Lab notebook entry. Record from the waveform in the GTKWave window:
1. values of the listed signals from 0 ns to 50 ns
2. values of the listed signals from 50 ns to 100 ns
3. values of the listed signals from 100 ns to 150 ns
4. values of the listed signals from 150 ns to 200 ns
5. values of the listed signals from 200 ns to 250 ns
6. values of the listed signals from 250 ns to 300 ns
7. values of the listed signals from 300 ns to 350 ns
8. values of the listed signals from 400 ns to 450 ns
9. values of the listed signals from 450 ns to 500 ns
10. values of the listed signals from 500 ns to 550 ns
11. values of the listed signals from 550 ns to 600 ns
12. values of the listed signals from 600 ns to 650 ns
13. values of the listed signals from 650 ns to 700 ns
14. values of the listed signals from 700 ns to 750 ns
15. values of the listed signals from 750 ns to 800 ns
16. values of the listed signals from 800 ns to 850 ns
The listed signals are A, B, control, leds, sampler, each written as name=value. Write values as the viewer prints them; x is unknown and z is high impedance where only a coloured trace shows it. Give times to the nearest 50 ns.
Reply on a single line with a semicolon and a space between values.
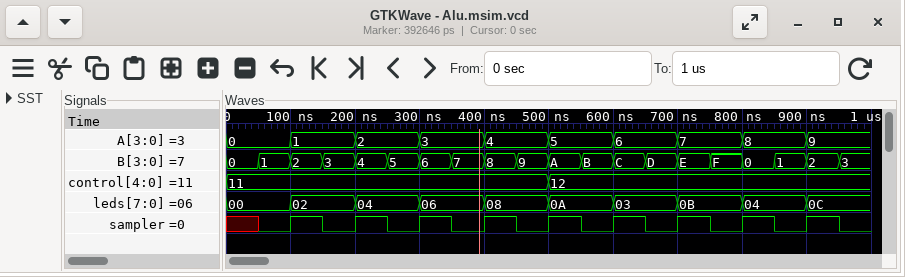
A=0, B=0, control=11, leds=00, sampler=x; A=0, B=1, control=11, leds=00, sampler=0; A=1, B=2, control=11, leds=02, sampler=1; A=1, B=3, control=11, leds=02, sampler=0; A=2, B=4, control=11, leds=04, sampler=1; A=2, B=5, control=11, leds=04, sampler=0; A=3, B=6, control=11, leds=06, sampler=1; A=4, B=8, control=11, leds=08, sampler=1; A=4, B=9, control=11, leds=08, sampler=0; A=5, B=A, control=12, leds=0A, sampler=1; A=5, B=B, control=12, leds=0A, sampler=0; A=6, B=C, control=12, leds=03, sampler=1; A=6, B=D, control=12, leds=03, sampler=0; A=7, B=E, control=12, leds=0B, sampler=1; A=7, B=F, control=12, leds=0B, sampler=0; A=8, B=0, control=12, leds=04, sampler=1
